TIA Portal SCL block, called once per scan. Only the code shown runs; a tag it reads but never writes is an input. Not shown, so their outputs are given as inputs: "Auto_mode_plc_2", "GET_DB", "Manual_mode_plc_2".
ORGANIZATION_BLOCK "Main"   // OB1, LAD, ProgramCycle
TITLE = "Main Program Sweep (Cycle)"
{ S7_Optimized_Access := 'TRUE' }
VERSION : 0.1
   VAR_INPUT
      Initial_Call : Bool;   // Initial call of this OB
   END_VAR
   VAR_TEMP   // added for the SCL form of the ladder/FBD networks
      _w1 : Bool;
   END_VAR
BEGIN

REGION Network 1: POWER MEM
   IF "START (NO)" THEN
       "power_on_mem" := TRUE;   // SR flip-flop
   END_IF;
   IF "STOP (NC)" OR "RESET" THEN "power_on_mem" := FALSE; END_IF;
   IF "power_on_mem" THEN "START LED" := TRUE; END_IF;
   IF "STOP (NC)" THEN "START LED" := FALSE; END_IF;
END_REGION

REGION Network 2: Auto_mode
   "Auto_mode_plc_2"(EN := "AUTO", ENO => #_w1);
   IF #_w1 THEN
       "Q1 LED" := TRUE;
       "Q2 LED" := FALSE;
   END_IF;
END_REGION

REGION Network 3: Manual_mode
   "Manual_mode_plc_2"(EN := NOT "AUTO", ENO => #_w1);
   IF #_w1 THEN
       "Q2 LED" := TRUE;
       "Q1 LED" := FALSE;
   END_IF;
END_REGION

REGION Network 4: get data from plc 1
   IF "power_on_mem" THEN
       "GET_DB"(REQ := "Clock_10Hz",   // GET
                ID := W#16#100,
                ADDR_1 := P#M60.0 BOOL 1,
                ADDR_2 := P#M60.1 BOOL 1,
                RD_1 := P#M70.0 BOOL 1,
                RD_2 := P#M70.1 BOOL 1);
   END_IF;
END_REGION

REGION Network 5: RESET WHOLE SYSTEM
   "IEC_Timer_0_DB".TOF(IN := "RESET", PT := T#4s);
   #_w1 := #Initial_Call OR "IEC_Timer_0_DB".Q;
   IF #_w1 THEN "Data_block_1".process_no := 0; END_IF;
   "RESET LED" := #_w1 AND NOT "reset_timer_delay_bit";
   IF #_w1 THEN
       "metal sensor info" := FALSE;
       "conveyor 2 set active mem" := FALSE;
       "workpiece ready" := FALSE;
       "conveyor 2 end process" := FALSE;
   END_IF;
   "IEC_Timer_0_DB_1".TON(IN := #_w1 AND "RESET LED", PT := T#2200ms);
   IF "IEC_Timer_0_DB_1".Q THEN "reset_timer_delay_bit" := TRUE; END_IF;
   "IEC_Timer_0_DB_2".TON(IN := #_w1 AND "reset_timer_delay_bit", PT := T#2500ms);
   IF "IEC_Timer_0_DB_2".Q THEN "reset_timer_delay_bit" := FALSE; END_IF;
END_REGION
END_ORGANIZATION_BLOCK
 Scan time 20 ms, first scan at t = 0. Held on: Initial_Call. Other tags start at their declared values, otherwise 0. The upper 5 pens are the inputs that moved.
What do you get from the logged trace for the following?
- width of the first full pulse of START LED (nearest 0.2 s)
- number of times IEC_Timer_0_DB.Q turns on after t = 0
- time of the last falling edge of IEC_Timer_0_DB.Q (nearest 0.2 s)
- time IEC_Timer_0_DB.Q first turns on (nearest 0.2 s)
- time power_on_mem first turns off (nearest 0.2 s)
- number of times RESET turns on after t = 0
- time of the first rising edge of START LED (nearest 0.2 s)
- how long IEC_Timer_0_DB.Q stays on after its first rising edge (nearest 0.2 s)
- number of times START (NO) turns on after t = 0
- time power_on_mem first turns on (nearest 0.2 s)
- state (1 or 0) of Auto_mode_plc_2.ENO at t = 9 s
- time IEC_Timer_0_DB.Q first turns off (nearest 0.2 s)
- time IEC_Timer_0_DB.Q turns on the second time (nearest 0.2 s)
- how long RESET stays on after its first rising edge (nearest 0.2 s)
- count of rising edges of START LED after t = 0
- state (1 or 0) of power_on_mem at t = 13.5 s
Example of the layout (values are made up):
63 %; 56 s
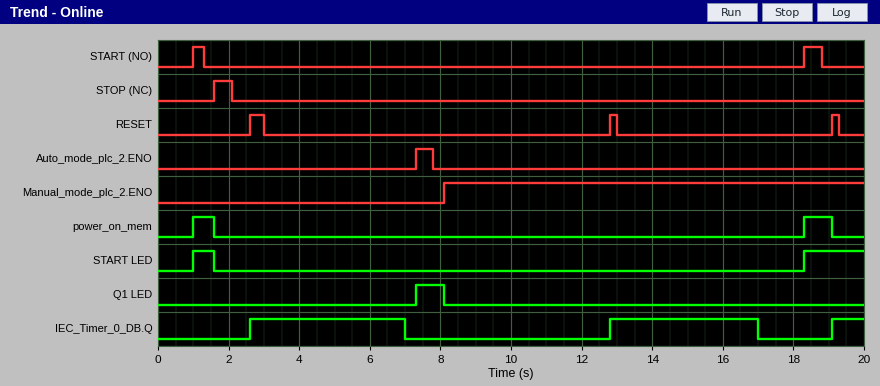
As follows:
0.6 s; 3; 17.0 s; 2.6 s; 1.6 s; 3; 1.0 s; 4.4 s; 2; 1.0 s; 0; 7.0 s; 12.8 s; 0.4 s; 2; 0
